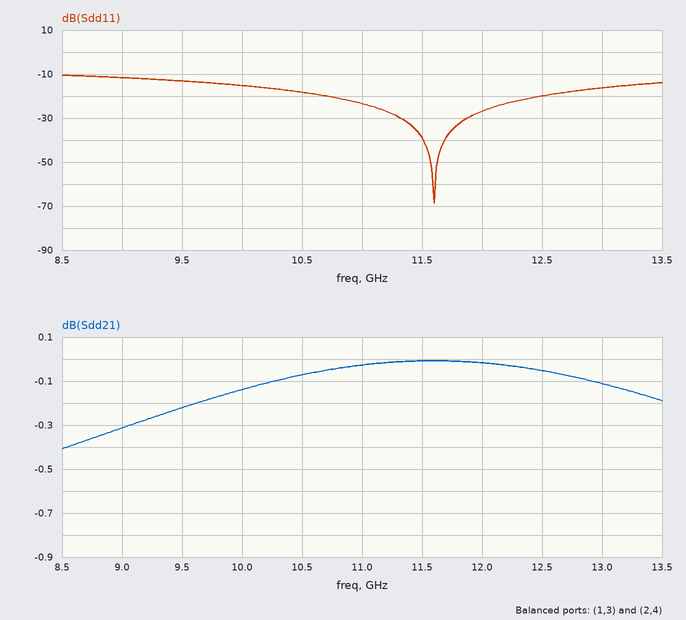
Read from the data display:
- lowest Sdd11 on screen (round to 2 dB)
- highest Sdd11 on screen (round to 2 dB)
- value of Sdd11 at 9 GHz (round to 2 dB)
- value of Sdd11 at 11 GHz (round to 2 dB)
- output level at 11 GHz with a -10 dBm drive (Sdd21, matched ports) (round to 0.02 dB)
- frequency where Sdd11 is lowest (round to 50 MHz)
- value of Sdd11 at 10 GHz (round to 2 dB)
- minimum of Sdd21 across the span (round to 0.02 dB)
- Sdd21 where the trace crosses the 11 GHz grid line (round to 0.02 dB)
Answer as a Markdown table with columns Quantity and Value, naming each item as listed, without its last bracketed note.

| Quantity | Value |
|---|---|
| lowest Sdd11 on screen | -68 dB |
| highest Sdd11 on screen | -10 dB |
| value of Sdd11 at 9 GHz | -12 dB |
| value of Sdd11 at 11 GHz | -24 dB |
| output level at 11 GHz with a -10 dBm drive (Sdd21, matched ports) | -10.02 dBm |
| frequency where Sdd11 is lowest | 11.60 GHz |
| value of Sdd11 at 10 GHz | -16 dB |
| minimum of Sdd21 across the span | -0.40 dB |
| Sdd21 where the trace crosses the 11 GHz grid line | -0.02 dB |
